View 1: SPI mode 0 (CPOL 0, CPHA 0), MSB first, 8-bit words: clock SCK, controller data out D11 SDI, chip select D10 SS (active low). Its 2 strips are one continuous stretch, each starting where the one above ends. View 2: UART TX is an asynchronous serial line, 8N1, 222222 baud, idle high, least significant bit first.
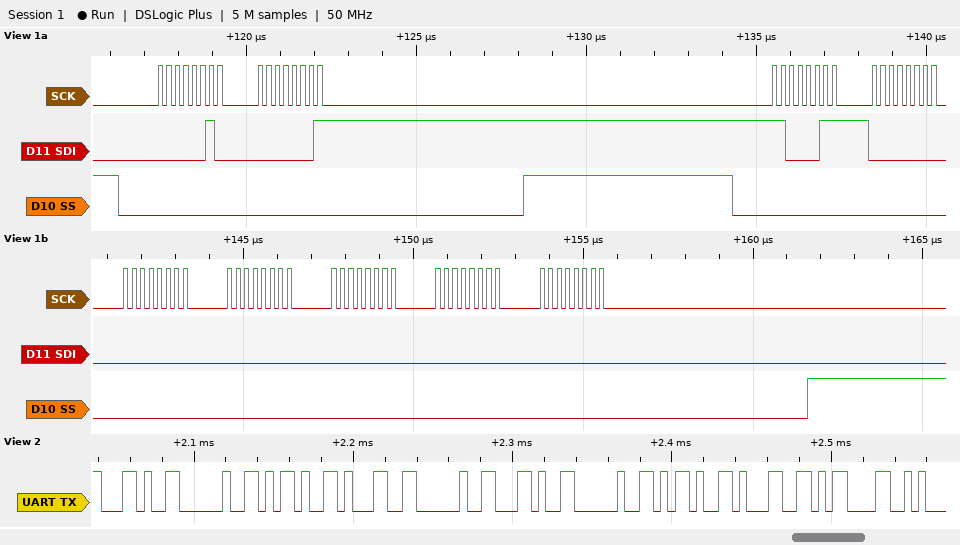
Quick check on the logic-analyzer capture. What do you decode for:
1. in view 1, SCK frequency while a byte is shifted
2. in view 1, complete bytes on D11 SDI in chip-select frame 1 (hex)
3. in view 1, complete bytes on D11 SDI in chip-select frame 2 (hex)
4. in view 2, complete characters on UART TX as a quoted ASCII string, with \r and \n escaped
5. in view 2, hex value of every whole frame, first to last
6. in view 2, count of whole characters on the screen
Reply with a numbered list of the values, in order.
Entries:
1. 4 MHz
2. 02 01
3. C3 00 00 00 00 00 00
4. ", -1 , -1\r"
5. 2C 20 2D 31 20 2C 20 2D 31 0D
6. 10
